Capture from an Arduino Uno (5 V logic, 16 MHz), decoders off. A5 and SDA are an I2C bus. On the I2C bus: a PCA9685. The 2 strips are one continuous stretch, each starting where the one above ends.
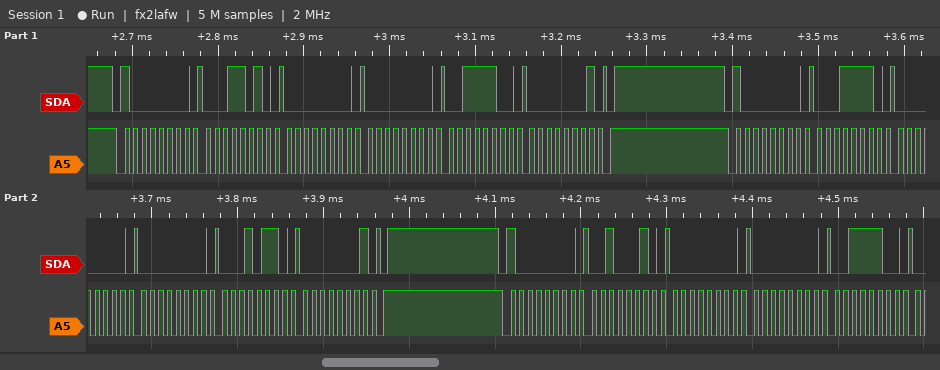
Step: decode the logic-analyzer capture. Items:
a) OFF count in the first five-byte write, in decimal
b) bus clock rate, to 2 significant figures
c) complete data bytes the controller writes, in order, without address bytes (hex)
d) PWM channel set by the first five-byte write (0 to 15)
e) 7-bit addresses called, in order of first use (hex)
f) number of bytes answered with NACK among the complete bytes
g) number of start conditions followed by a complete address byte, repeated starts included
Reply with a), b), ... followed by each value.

a) 316
b) 100 kHz
c) 1A 00 00 3C 01 1E 00 00 16 01 22 00 00 3C
d) 5
e) 0x40
f) 0
g) 3
